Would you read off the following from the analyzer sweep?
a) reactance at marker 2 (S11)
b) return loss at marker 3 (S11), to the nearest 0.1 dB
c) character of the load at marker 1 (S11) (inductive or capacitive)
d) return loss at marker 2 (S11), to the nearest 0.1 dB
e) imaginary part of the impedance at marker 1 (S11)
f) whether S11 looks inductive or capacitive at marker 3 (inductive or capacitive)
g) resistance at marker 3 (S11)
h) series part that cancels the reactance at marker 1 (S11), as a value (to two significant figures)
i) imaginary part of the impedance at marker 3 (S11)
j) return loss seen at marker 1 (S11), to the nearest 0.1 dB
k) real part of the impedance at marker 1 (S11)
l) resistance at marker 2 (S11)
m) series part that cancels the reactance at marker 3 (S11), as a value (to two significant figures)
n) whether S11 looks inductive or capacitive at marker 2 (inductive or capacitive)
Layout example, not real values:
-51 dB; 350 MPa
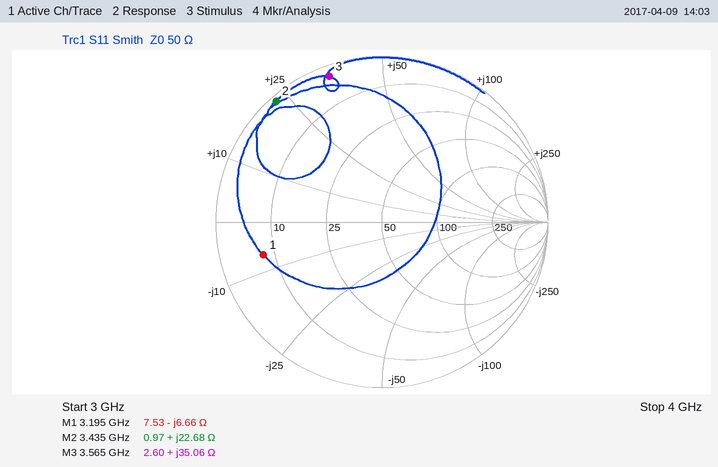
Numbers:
+22.68 Ω; 0.6 dB; capacitive; 0.3 dB; -6.66 Ω; inductive; 2.60 Ω; 330 pH; +35.06 Ω; 2.6 dB; 7.53 Ω; 0.97 Ω; 1.3 pF; inductive
